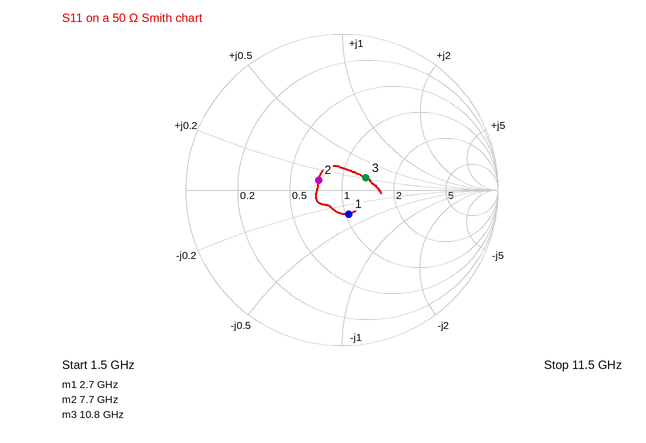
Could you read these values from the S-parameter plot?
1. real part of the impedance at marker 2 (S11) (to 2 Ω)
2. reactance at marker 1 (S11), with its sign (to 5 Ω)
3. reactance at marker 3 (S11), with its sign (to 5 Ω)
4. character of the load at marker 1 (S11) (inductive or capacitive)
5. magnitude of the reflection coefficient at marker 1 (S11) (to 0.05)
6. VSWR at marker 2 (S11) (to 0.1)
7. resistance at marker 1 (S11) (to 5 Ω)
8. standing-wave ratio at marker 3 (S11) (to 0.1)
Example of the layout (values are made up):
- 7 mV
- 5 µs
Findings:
- 36 Ω
- -15 Ω
- +10 Ω
- capacitive
- 0.15
- 1.4
- 50 Ω
- 1.4
